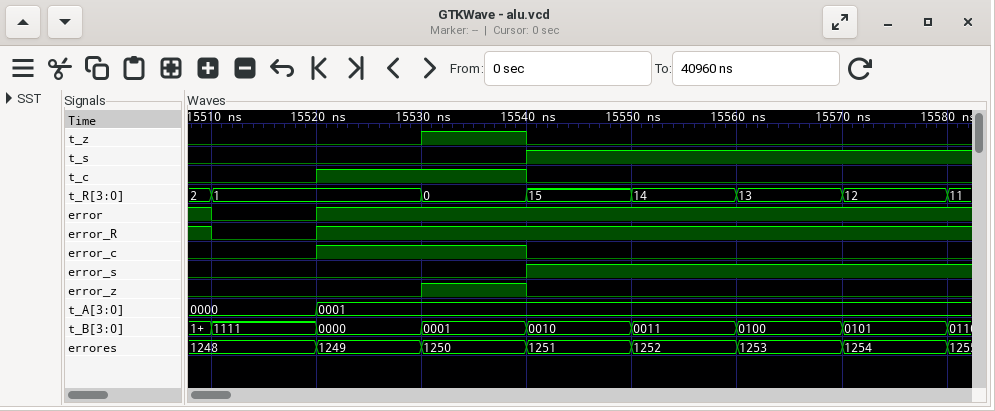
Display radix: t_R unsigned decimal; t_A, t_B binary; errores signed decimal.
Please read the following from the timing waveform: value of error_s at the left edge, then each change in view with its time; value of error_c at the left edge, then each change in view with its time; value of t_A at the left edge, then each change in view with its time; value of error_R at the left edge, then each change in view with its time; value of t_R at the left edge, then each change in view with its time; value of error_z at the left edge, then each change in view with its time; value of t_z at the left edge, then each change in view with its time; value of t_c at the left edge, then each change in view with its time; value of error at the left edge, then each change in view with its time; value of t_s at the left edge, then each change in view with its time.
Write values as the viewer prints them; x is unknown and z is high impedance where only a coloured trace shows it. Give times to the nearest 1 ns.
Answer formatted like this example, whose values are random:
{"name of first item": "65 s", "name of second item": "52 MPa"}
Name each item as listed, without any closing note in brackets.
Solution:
{"value of error_s at the left edge, then each change in view with its time": "0, 1 at 15540 ns", "value of error_c at the left edge, then each change in view with its time": "0, 1 at 15520 ns, 0 at 15540 ns", "value of t_A at the left edge, then each change in view with its time": "0000, 0001 at 15520 ns", "value of error_R at the left edge, then each change in view with its time": "1, 0 at 15510 ns, 1 at 15520 ns", "value of t_R at the left edge, then each change in view with its time": "2, 1 at 15510 ns, 0 at 15530 ns, 15 at 15540 ns, 14 at 15550 ns, 13 at 15560 ns, 12 at 15570 ns, 11 at 15580 ns", "value of error_z at the left edge, then each change in view with its time": "0, 1 at 15530 ns, 0 at 15540 ns", "value of t_z at the left edge, then each change in view with its time": "0, 1 at 15530 ns, 0 at 15540 ns", "value of t_c at the left edge, then each change in view with its time": "0, 1 at 15520 ns, 0 at 15540 ns", "value of error at the left edge, then each change in view with its time": "1, 0 at 15510 ns, 1 at 15520 ns", "value of t_s at the left edge, then each change in view with its time": "0, 1 at 15540 ns"}
